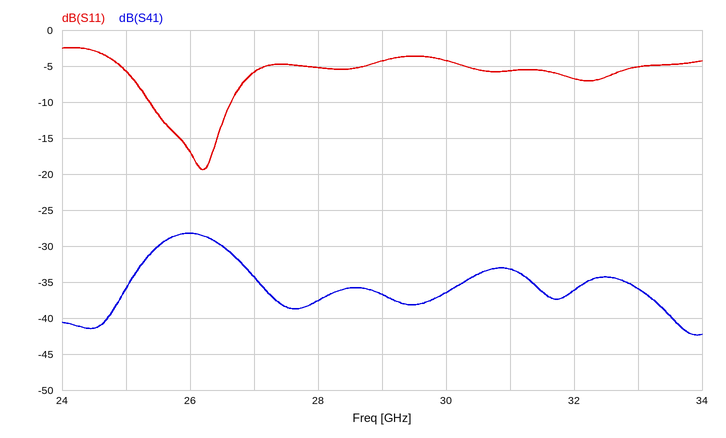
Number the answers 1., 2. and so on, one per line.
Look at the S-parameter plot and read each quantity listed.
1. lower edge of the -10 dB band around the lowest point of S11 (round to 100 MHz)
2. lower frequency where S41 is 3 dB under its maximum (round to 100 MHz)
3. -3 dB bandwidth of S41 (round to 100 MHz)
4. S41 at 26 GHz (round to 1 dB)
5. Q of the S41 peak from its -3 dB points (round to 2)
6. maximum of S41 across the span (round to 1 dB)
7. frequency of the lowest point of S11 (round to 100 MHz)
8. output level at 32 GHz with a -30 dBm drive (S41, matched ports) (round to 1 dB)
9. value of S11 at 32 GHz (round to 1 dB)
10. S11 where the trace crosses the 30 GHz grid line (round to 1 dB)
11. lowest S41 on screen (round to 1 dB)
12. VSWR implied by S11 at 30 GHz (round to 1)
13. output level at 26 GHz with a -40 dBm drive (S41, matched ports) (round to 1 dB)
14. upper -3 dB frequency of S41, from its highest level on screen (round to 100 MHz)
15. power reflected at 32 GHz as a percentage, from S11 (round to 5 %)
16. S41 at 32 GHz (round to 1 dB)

1. 25.4 GHz
2. 25.4 GHz
3. 1.3 GHz
4. -28 dB
5. 20
6. -28 dB
7. 26.2 GHz
8. -66 dBm
9. -7 dB
10. -4 dB
11. -42 dB
12. 4
13. -68 dBm
14. 26.7 GHz
15. 20 %
16. -36 dB
